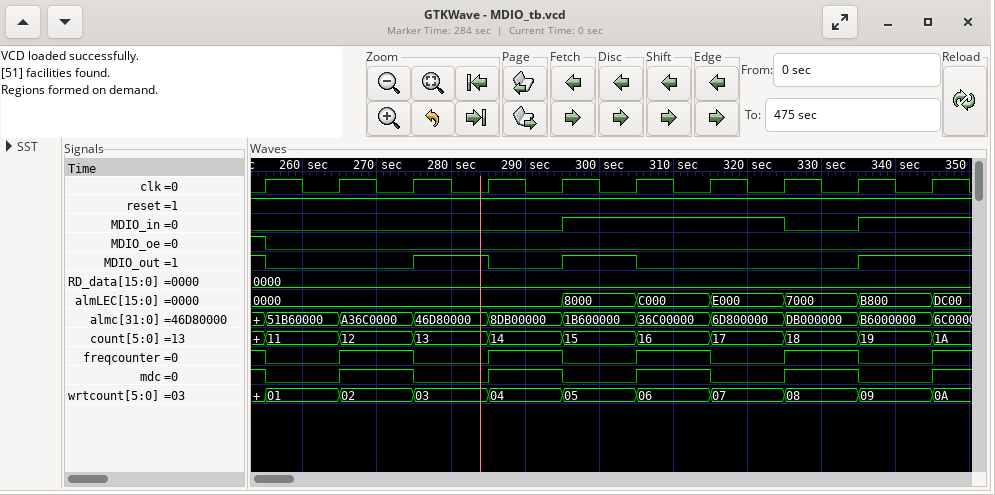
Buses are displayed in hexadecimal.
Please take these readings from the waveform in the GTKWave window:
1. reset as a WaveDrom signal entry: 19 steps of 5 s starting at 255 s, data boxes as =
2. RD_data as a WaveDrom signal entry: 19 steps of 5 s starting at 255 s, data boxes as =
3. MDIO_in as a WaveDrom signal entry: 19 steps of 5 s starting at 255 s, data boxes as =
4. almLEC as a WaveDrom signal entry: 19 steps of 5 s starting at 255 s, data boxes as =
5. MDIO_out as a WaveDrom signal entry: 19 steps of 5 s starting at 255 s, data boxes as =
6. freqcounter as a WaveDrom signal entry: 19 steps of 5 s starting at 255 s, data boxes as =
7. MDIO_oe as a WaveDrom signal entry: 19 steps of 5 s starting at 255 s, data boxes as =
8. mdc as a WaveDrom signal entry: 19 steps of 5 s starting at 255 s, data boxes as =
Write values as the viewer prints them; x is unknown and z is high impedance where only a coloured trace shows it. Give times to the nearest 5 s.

{name: 'reset', wave: '1..................'}
{name: 'RD_data', wave: '=..................', data: '0000'}
{name: 'MDIO_in', wave: '0.......1.....0.1..'}
{name: 'almLEC', wave: '=.......=.=.=.=.=.=', data: '0000 8000 C000 E000 7000 B800 DC00'}
{name: 'MDIO_out', wave: '0...1.0.1.0.....1..'}
{name: 'freqcounter', wave: '0.1.0.1.0.1.0.1.0.1'}
{name: 'MDIO_oe', wave: '0..................'}
{name: 'mdc', wave: '0.1.0.1.0.1.0.1.0.1'}
